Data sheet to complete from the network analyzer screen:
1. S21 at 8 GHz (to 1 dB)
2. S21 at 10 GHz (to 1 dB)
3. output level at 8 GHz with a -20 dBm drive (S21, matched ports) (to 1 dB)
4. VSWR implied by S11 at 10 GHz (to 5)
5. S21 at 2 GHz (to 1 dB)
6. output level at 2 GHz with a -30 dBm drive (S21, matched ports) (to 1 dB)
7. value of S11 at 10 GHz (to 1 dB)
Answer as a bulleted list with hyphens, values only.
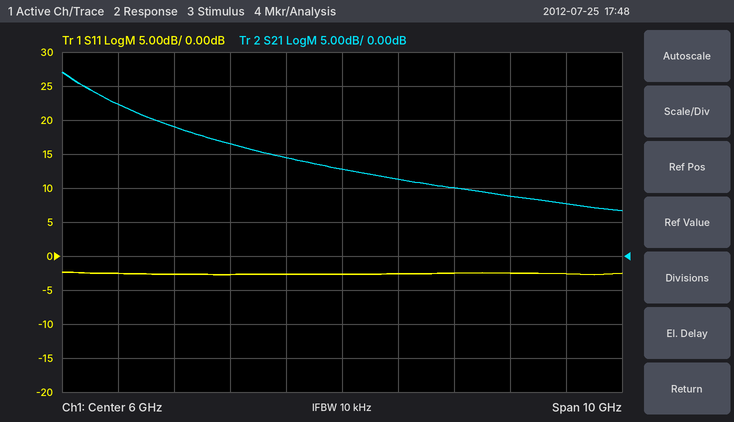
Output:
- 10 dB
- 8 dB
- -10 dBm
- 5
- 22 dB
- -8 dBm
- -3 dB
